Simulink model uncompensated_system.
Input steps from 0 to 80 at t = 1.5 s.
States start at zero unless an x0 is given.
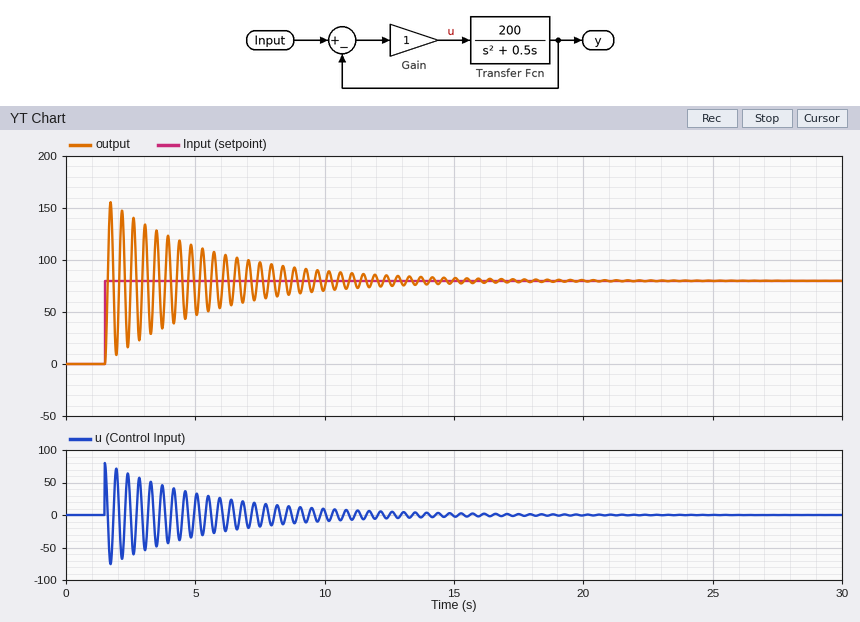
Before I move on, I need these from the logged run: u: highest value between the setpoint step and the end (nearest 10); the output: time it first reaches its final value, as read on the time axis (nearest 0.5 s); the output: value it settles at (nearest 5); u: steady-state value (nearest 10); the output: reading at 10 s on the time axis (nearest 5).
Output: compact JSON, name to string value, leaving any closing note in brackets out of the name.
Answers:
{"u: highest value between the setpoint step and the end": "80", "the output: time it first reaches its final value, as read on the time axis": "1.5 s", "the output: value it settles at": "80", "u: steady-state value": "0", "the output: reading at 10 s on the time axis": "75"}
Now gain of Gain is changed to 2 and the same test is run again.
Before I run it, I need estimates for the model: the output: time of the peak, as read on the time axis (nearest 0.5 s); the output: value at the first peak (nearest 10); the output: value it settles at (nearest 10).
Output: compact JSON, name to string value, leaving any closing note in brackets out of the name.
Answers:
{"the output: time of the peak, as read on the time axis": "1.5 s", "the output: value at the first peak": "160", "the output: value it settles at": "80"}
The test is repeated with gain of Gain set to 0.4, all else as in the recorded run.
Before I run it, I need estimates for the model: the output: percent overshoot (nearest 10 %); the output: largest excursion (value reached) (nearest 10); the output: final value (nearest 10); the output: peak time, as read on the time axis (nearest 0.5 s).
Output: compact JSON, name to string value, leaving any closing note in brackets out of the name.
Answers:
{"the output: percent overshoot": "90 %", "the output: largest excursion (value reached)": "150", "the output: final value": "80", "the output: peak time, as read on the time axis": "2.0 s"}
